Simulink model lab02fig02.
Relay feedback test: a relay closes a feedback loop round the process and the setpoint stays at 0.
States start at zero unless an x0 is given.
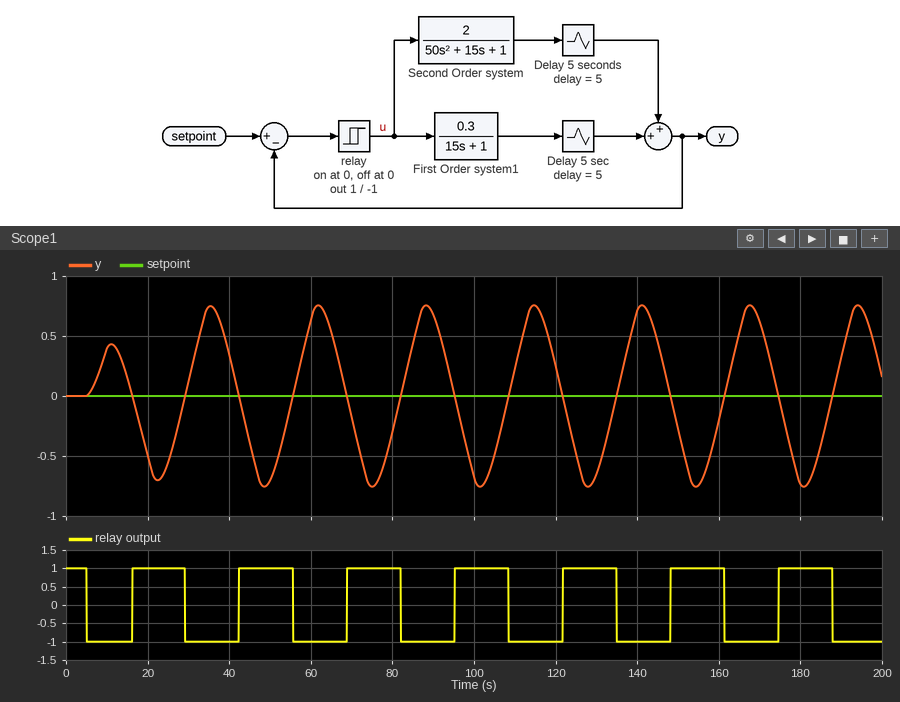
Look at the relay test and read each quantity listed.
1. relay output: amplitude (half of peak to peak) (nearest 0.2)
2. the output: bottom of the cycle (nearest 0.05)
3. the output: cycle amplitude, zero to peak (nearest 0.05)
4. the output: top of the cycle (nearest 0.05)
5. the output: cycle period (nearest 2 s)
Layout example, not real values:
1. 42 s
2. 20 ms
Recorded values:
1. 1.0
2. -0.75
3. 0.75
4. 0.75
5. 26 s
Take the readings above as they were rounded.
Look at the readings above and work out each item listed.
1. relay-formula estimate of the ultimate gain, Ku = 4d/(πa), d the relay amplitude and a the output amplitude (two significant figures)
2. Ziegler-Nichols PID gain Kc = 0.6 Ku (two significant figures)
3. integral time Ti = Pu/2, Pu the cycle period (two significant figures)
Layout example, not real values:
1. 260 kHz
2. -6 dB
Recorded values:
1. 1.7
2. 1.0
3. 13 s
